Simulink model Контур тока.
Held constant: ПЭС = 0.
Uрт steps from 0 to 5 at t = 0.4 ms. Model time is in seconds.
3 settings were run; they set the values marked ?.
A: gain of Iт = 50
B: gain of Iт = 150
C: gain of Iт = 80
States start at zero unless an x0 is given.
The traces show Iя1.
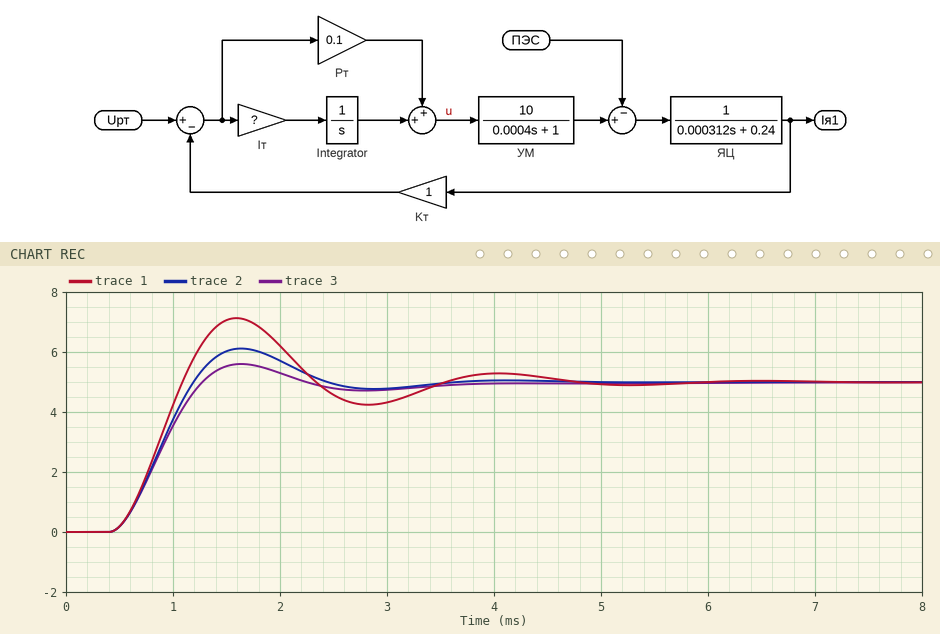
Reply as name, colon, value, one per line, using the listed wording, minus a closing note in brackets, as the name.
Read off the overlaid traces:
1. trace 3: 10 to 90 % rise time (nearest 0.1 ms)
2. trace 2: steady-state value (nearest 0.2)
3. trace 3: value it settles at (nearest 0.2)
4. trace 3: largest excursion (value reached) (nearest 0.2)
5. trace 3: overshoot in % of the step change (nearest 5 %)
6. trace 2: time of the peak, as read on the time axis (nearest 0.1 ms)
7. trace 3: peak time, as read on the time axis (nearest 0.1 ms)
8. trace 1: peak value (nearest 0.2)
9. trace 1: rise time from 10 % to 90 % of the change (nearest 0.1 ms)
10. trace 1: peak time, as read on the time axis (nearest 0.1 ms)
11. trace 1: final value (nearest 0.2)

trace 3: 10 to 90 % rise time: 0.6 ms
trace 2: steady-state value: 5.0
trace 3: value it settles at: 5.0
trace 3: largest excursion (value reached): 5.6
trace 3: overshoot in % of the step change: 10 %
trace 2: time of the peak, as read on the time axis: 1.6 ms
trace 3: peak time, as read on the time axis: 1.6 ms
trace 1: peak value: 7.2
trace 1: rise time from 10 % to 90 % of the change: 0.5 ms
trace 1: peak time, as read on the time axis: 1.6 ms
trace 1: final value: 5.0
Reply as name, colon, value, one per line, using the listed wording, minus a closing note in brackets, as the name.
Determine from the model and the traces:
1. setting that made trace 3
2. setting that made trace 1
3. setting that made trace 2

setting that made trace 3: A
setting that made trace 1: B
setting that made trace 2: C
